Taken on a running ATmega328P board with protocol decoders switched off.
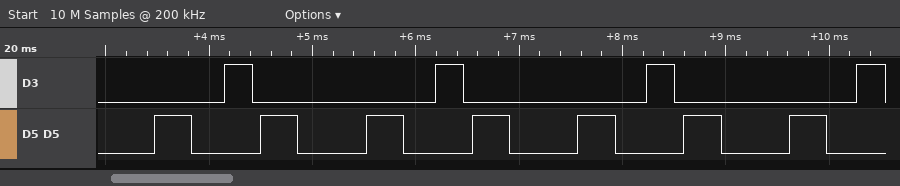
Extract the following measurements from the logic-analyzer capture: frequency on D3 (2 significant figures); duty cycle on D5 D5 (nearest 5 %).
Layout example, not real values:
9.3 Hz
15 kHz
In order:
490 Hz
35 %
